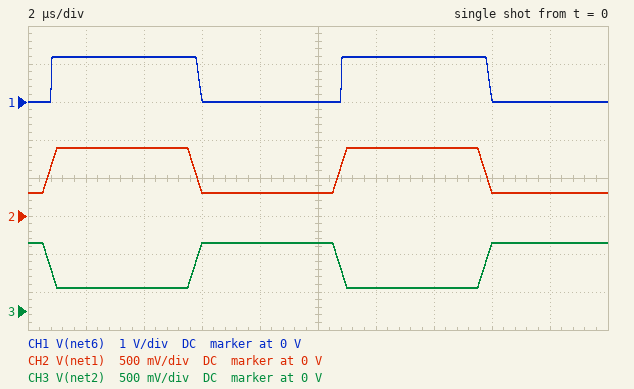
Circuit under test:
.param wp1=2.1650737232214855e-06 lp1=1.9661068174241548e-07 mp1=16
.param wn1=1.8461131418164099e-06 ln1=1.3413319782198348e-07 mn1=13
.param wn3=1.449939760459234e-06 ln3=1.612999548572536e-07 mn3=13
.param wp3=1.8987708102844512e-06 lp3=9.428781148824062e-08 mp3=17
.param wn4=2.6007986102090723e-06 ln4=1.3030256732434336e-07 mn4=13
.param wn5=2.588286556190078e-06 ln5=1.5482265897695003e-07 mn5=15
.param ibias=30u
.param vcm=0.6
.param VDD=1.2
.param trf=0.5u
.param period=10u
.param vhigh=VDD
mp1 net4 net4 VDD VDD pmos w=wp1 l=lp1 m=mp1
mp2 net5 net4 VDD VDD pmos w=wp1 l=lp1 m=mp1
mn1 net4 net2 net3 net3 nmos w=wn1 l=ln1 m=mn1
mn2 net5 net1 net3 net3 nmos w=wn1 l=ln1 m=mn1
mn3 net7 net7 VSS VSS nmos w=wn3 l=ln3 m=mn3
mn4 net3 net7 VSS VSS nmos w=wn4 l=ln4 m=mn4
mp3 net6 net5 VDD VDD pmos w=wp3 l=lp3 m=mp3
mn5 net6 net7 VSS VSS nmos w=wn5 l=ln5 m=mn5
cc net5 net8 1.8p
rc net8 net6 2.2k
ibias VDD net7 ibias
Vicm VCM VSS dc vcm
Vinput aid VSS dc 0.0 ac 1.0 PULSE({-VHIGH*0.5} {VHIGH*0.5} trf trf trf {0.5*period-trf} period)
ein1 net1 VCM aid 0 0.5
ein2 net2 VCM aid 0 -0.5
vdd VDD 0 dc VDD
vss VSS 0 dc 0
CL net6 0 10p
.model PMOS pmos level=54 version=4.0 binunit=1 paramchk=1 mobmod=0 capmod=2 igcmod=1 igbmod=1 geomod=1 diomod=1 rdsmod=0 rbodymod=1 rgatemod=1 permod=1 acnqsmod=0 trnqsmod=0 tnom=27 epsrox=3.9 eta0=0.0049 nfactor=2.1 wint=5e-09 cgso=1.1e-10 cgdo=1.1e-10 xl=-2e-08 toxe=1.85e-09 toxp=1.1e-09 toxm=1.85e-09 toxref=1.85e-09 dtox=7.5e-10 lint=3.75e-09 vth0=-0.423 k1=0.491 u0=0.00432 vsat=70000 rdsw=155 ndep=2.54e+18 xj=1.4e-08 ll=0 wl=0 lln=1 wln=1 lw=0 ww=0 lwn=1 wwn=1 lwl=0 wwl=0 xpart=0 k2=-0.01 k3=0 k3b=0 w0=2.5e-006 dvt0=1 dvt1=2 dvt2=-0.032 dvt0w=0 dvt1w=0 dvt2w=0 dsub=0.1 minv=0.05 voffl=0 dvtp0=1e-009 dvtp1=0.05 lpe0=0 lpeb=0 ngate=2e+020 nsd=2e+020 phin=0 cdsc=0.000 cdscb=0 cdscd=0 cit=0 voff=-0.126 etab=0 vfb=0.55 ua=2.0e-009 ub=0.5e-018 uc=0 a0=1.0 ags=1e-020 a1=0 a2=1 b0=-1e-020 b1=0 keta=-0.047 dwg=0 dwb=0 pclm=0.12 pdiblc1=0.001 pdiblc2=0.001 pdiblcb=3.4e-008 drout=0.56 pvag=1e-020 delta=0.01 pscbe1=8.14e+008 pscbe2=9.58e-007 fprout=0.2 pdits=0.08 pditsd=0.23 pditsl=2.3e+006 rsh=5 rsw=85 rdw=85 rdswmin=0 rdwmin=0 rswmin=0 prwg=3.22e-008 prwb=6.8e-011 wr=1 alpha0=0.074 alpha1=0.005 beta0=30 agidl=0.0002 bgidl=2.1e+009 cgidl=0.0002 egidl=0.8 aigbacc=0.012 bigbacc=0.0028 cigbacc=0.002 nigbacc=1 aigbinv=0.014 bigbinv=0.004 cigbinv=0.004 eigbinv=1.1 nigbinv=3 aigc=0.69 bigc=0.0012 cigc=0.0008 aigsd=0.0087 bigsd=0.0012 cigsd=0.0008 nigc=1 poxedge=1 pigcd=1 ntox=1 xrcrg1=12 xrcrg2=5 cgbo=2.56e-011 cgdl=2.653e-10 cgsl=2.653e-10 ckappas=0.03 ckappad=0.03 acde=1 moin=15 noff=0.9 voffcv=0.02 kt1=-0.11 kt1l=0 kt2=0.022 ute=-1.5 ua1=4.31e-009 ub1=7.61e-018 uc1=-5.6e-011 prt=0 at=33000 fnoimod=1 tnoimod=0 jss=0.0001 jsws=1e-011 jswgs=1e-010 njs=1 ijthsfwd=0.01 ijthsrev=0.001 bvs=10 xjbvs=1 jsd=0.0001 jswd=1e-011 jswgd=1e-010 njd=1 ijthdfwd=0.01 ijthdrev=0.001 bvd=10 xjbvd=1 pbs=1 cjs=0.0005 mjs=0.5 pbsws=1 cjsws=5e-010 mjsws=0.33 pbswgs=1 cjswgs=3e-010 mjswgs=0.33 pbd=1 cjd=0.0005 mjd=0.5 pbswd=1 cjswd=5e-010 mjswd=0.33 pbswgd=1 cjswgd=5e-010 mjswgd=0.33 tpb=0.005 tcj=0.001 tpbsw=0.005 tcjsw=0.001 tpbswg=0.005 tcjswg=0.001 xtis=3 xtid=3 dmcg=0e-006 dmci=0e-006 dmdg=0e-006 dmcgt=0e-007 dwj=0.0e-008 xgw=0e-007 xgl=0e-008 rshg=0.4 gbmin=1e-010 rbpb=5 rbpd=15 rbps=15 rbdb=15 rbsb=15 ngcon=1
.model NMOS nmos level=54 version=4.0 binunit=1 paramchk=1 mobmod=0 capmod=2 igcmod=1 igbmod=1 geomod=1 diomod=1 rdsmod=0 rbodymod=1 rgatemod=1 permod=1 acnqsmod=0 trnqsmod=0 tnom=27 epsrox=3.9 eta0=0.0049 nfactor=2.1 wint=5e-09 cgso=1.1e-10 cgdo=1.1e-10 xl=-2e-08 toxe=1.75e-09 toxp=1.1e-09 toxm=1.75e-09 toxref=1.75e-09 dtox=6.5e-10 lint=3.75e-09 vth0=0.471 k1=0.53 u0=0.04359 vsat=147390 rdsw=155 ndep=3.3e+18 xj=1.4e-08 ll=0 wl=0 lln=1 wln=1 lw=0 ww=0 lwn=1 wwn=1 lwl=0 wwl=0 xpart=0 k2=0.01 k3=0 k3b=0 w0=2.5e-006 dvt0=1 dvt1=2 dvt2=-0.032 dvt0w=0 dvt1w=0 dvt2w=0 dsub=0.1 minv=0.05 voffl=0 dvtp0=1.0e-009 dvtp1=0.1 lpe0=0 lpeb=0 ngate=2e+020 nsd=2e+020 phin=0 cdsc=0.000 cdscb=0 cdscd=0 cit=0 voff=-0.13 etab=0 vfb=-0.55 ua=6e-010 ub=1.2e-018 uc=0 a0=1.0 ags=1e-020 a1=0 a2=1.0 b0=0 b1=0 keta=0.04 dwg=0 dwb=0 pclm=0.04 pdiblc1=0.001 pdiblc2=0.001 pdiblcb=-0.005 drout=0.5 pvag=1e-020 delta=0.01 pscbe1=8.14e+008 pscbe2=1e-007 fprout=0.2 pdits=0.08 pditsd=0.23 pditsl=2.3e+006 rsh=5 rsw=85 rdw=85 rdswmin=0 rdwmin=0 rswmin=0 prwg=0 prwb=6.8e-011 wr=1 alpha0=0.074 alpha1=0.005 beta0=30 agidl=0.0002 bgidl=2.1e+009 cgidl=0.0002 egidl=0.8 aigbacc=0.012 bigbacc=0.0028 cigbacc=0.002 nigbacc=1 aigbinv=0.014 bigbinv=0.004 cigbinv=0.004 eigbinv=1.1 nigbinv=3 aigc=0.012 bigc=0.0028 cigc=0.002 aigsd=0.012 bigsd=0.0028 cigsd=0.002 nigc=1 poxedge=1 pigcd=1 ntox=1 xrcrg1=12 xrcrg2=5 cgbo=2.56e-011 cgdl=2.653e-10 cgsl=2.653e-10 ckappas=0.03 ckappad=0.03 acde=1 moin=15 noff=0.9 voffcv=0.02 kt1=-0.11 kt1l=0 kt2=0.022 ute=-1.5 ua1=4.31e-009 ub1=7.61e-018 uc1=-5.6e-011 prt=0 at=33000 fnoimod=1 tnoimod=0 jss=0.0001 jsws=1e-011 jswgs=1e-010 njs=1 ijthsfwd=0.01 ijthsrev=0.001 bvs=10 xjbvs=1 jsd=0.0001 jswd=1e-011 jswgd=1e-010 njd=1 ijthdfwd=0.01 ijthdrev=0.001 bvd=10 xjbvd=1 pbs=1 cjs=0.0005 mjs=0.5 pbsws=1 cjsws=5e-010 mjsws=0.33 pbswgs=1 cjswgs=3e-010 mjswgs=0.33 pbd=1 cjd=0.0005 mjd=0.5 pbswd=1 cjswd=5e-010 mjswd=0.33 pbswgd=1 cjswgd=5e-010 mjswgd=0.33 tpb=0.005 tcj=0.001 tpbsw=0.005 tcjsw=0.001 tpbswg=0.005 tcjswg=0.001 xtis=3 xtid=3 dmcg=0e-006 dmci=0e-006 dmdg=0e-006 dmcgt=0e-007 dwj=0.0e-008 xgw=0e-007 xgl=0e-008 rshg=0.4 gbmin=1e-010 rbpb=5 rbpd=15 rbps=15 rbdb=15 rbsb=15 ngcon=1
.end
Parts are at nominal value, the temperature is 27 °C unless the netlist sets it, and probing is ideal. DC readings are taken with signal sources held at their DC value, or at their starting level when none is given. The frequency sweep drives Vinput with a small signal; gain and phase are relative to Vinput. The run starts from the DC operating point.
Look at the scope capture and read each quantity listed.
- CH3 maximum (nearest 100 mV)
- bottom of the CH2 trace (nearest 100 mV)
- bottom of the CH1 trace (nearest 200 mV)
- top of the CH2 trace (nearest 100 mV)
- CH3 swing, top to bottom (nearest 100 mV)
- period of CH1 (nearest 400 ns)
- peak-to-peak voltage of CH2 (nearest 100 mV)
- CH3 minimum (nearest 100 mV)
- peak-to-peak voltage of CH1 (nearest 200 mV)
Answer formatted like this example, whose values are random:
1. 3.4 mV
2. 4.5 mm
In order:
1. 900 mV
2. 300 mV
3. 0 V
4. 900 mV
5. 600 mV
6. 10.0 µs
7. 600 mV
8. 300 mV
9. 1.2 V
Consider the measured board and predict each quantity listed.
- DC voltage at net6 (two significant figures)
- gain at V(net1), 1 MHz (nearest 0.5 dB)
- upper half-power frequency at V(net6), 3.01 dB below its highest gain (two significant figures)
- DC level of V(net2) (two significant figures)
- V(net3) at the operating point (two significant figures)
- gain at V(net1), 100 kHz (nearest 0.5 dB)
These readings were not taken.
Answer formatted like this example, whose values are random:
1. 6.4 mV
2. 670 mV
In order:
1. 1.1 V
2. -6.0 dB
3. 170 kHz
4. 600 mV
5. 220 mV
6. -6.0 dB
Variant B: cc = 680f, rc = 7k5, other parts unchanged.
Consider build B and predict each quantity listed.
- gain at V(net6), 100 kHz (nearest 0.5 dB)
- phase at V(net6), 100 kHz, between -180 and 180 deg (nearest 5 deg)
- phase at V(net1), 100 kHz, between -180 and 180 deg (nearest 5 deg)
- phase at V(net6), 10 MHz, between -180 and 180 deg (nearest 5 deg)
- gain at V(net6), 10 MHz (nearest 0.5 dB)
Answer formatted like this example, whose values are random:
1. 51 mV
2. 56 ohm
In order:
1. 48.0 dB
2. -15 deg
3. 0 deg
4. -100 deg
5. 20.0 dB
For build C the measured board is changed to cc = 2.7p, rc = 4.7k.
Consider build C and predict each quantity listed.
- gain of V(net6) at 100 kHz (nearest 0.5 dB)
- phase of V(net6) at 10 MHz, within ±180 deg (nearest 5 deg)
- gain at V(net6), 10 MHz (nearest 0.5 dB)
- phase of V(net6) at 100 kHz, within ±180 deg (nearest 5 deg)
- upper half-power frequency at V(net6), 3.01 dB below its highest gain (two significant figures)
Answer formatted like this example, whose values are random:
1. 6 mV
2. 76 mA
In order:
1. 46.0 dB
2. -85 deg
3. 10.0 dB
4. -40 deg
5. 110 kHz
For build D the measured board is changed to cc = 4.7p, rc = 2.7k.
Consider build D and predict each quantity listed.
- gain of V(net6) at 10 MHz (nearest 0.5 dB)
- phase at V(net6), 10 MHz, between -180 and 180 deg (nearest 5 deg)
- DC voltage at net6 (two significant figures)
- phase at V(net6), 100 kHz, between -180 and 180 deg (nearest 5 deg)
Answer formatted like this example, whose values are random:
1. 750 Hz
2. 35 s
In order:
1. 5.0 dB
2. -90 deg
3. 1.1 V
4. -55 deg
